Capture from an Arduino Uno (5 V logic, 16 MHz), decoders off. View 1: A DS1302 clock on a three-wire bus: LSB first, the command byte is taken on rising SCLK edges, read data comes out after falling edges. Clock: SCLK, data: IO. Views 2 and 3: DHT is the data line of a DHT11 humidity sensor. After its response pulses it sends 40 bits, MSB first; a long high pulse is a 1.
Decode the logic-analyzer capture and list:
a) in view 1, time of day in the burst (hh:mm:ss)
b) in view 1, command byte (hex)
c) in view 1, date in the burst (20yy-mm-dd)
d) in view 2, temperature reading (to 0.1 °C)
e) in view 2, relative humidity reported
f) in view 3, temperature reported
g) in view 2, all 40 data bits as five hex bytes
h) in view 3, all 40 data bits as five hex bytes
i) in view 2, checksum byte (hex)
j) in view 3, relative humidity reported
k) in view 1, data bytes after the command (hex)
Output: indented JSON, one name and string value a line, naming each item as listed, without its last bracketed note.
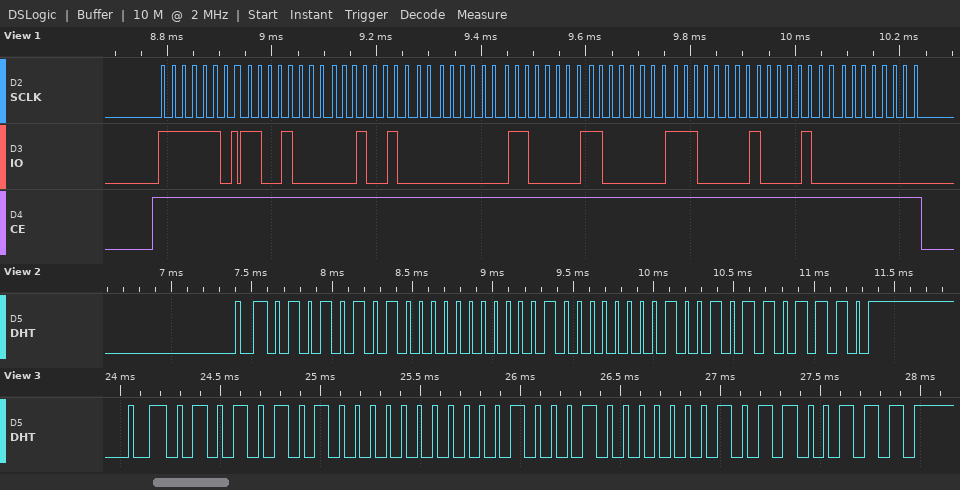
{
  "in view 1, time of day in the burst": "00:48:13",
  "in view 1, command byte": "0xBF",
  "in view 1, date in the burst": "2021-03-06",
  "in view 2, temperature reading": "16.9 °C",
  "in view 2, relative humidity reported": "85 %",
  "in view 3, temperature reported": "17.1 °C",
  "in view 2, all 40 data bits as five hex bytes": "55 00 10 09 6E",
  "in view 3, all 40 data bits as five hex bytes": "55 00 11 01 67",
  "in view 2, checksum byte": "0x6E",
  "in view 3, relative humidity reported": "85 %",
  "in view 1, data bytes after the command": "13 48 00 06 03 07 21 00"
}
